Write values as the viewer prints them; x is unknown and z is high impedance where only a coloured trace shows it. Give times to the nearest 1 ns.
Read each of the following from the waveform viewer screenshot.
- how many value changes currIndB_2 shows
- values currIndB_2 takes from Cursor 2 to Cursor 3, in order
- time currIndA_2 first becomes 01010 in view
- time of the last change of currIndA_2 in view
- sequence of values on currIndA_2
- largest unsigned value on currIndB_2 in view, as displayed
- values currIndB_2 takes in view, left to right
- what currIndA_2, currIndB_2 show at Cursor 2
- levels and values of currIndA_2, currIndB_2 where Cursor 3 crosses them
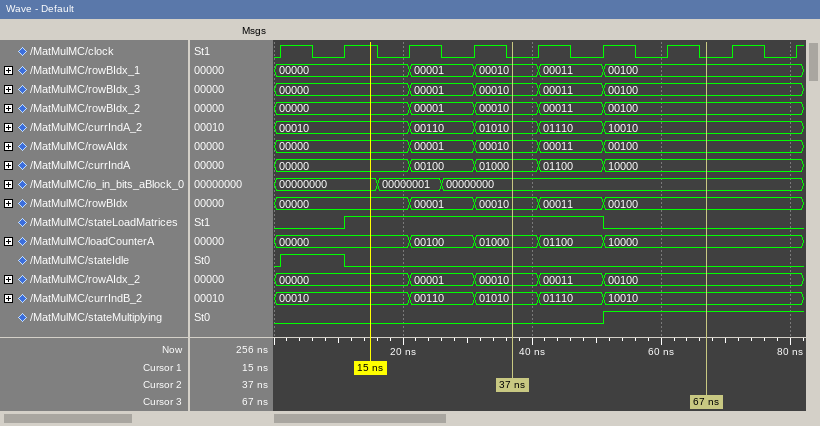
4
01010, 01110, 10010
31 ns
51 ns
00010, 00110, 01010, 01110, 10010
10010
00010, 00110, 01010, 01110, 10010
currIndA_2=01010, currIndB_2=01010
currIndA_2=10010, currIndB_2=10010
